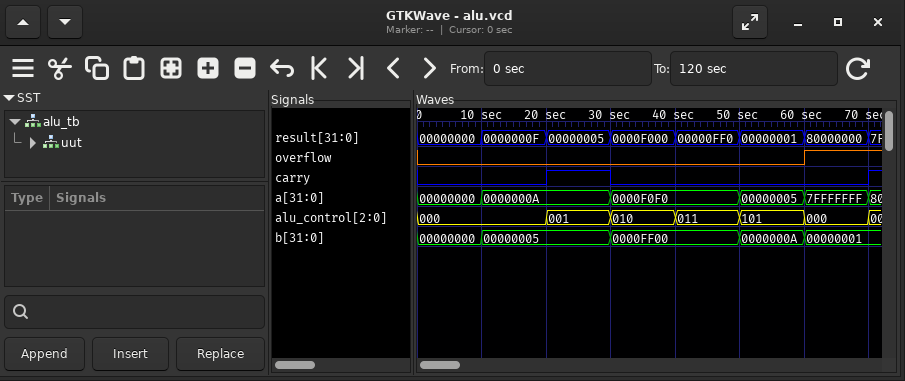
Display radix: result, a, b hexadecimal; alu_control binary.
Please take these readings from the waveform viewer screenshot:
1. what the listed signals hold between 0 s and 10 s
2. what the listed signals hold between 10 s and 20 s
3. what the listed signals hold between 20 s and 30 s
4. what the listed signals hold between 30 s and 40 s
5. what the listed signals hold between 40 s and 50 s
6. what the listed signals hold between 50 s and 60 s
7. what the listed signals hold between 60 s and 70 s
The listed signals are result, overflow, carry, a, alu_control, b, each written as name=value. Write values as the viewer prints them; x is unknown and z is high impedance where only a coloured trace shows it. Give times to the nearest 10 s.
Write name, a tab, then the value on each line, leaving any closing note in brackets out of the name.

what the listed signals hold between 0 s and 10 s	result=00000000, overflow=0, carry=0, a=00000000, alu_control=000, b=00000000
what the listed signals hold between 10 s and 20 s	result=0000000F, overflow=0, carry=0, a=0000000A, alu_control=000, b=00000005
what the listed signals hold between 20 s and 30 s	result=00000005, overflow=0, carry=1, a=0000000A, alu_control=001, b=00000005
what the listed signals hold between 30 s and 40 s	result=0000F000, overflow=0, carry=0, a=0000F0F0, alu_control=010, b=0000FF00
what the listed signals hold between 40 s and 50 s	result=00000FF0, overflow=0, carry=0, a=0000F0F0, alu_control=011, b=0000FF00
what the listed signals hold between 50 s and 60 s	result=00000001, overflow=0, carry=0, a=00000005, alu_control=101, b=0000000A
what the listed signals hold between 60 s and 70 s	result=80000000, overflow=1, carry=0, a=7FFFFFFF, alu_control=000, b=00000001
